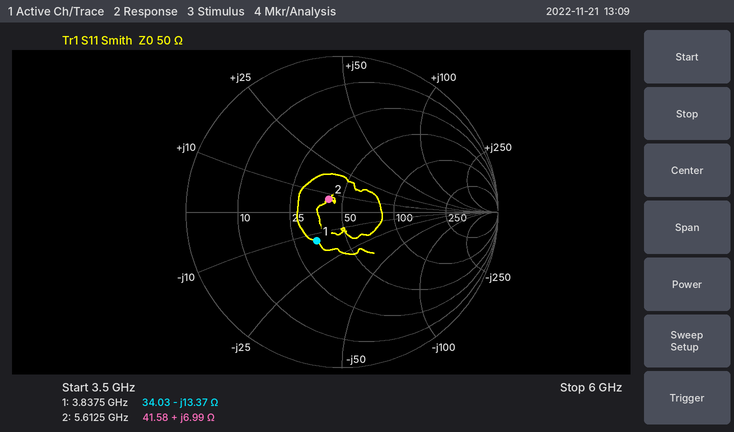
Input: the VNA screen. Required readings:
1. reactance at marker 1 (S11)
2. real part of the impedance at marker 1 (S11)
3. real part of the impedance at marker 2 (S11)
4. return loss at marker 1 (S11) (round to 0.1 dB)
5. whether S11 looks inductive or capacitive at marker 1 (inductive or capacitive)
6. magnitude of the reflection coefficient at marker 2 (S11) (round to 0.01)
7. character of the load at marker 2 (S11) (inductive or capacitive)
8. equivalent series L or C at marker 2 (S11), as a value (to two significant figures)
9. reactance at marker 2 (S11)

-13.37 Ω
34.03 Ω
41.58 Ω
12.2 dB
capacitive
0.12
inductive
200 pH
+6.99 Ω
